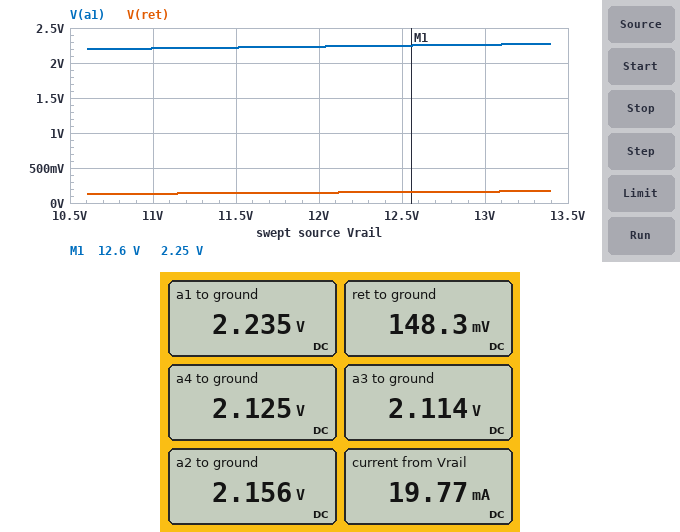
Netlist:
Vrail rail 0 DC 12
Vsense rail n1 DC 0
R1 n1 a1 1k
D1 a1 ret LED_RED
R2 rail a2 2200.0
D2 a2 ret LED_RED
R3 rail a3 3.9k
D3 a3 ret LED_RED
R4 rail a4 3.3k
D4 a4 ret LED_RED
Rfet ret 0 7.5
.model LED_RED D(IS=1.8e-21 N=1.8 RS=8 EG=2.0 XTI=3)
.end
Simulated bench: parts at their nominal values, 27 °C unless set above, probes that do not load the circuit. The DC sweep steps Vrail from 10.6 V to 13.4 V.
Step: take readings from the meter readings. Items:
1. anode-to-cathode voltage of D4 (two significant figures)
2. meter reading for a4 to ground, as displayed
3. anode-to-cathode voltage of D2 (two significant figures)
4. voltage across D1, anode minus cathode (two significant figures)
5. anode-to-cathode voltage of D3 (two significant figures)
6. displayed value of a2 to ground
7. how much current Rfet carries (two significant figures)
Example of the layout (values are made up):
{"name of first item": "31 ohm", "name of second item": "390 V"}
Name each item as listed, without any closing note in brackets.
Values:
{"anode-to-cathode voltage of D4": "2.0 V", "meter reading for a4 to ground, as displayed": "2.125 V", "anode-to-cathode voltage of D2": "2.0 V", "voltage across D1, anode minus cathode": "2.1 V", "anode-to-cathode voltage of D3": "2.0 V", "displayed value of a2 to ground": "2.156 V", "how much current Rfet carries": "20 mA"}
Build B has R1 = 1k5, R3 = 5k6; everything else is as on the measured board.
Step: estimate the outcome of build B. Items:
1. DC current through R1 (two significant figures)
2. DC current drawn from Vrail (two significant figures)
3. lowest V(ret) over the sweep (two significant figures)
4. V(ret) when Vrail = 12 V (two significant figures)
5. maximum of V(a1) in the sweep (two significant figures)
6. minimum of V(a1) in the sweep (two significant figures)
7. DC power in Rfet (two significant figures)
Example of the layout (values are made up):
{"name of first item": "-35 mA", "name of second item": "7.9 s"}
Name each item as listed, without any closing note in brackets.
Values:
{"DC current through R1": "6.6 mA", "DC current drawn from Vrail": "16 mA", "lowest V(ret) over the sweep": "100 mV", "V(ret) when Vrail = 12 V": "120 mV", "maximum of V(a1) in the sweep": "2.2 V", "minimum of V(a1) in the sweep": "2.1 V", "DC power in Rfet": "1.9 mW"}
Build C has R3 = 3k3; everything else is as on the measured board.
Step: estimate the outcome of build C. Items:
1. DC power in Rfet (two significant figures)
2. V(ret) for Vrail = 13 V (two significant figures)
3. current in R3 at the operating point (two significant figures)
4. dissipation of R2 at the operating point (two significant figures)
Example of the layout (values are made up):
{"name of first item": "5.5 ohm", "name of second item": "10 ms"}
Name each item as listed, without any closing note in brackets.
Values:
{"DC power in Rfet": "3.1 mW", "V(ret) for Vrail = 13 V": "170 mV", "current in R3 at the operating point": "3.0 mA", "dissipation of R2 at the operating point": "44 mW"}
